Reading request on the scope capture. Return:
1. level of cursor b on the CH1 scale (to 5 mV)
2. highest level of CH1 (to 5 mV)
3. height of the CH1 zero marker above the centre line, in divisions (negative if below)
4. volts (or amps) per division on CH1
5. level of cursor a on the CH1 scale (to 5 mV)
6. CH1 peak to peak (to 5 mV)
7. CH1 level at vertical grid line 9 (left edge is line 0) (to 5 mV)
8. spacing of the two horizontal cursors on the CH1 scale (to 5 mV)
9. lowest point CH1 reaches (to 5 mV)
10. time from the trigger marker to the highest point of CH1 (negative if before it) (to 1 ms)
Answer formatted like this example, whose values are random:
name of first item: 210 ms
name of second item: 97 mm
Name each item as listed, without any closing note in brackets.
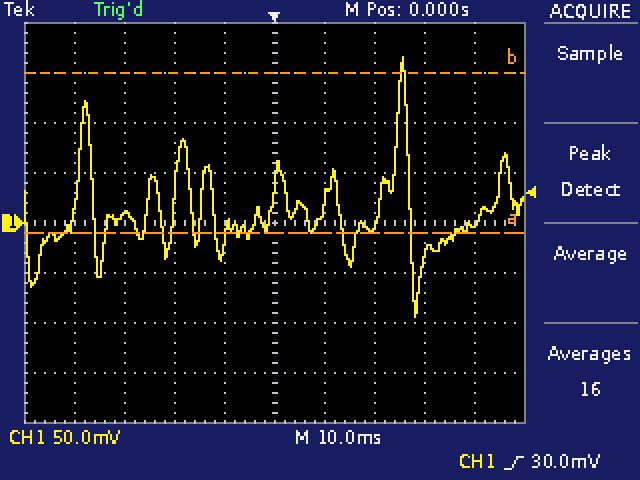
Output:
level of cursor b on the CH1 scale: 150 mV
highest level of CH1: 165 mV
height of the CH1 zero marker above the centre line, in divisions: 0.0 div
volts (or amps) per division on CH1: 50 mV
level of cursor a on the CH1 scale: -10 mV
CH1 peak to peak: 260 mV
CH1 level at vertical grid line 9 (left edge is line 0): 0 mV
spacing of the two horizontal cursors on the CH1 scale: 160 mV
lowest point CH1 reaches: -95 mV
time from the trigger marker to the highest point of CH1 (negative if before it): +26 ms
